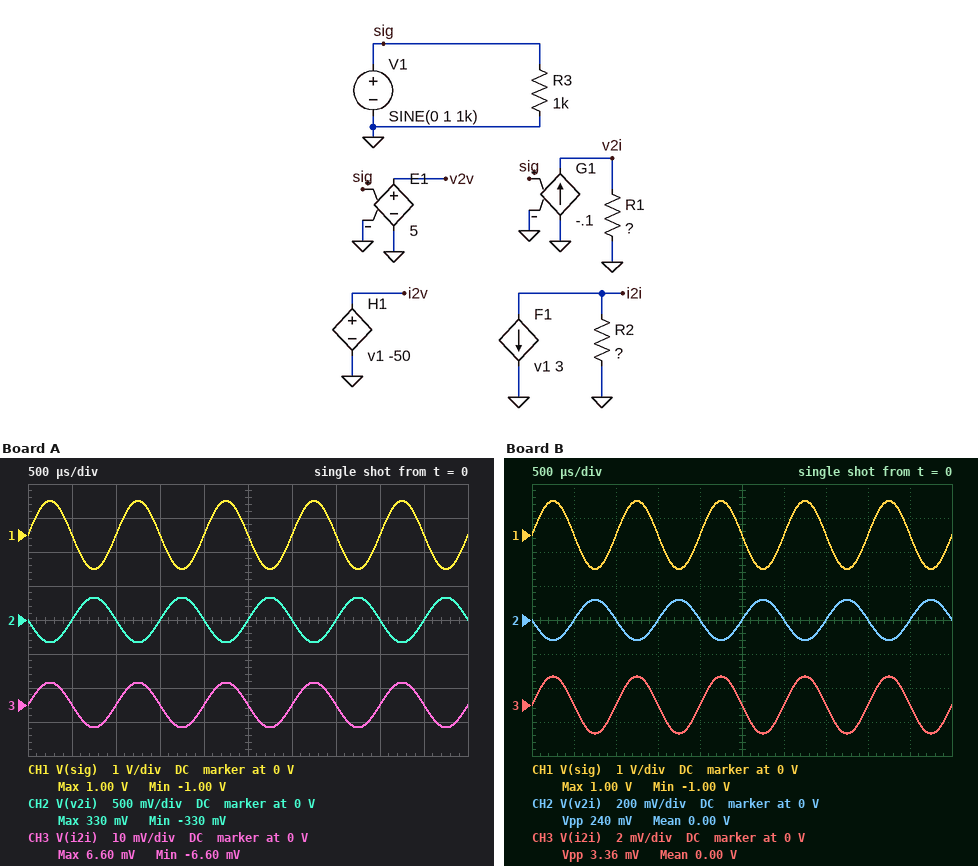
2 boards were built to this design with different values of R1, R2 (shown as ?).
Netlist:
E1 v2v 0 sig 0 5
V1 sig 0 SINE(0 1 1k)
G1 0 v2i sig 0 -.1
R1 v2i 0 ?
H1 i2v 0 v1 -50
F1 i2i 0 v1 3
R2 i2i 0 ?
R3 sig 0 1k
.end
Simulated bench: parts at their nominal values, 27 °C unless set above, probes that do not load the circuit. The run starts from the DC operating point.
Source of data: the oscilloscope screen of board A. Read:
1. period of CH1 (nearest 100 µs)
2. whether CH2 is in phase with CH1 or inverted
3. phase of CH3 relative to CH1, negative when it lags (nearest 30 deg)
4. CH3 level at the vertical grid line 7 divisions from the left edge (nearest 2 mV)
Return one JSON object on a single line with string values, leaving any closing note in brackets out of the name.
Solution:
{"period of CH1": "1.0 ms", "whether CH2 is in phase with CH1 or inverted": "inverted", "phase of CH3 relative to CH1, negative when it lags": "0 deg", "CH3 level at the vertical grid line 7 divisions from the left edge": "0 V"}
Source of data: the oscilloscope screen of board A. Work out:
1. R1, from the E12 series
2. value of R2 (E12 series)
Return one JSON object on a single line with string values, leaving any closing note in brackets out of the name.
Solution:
{"R1, from the E12 series": "3.3 Ω", "value of R2": "2.2 Ω"}
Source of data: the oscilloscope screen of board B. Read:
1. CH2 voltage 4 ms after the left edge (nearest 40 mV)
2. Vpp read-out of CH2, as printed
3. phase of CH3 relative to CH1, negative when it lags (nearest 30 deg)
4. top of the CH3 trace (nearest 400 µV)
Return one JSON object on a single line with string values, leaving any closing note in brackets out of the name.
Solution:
{"CH2 voltage 4 ms after the left edge": "0 V", "Vpp read-out of CH2, as printed": "240 mV", "phase of CH3 relative to CH1, negative when it lags": "0 deg", "top of the CH3 trace": "1.6 mV"}
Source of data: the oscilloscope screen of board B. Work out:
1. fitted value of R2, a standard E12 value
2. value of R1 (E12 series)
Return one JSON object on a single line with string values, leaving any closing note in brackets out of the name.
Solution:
{"fitted value of R2, a standard E12 value": "0.56 Ω", "value of R1": "1.2 Ω"}
